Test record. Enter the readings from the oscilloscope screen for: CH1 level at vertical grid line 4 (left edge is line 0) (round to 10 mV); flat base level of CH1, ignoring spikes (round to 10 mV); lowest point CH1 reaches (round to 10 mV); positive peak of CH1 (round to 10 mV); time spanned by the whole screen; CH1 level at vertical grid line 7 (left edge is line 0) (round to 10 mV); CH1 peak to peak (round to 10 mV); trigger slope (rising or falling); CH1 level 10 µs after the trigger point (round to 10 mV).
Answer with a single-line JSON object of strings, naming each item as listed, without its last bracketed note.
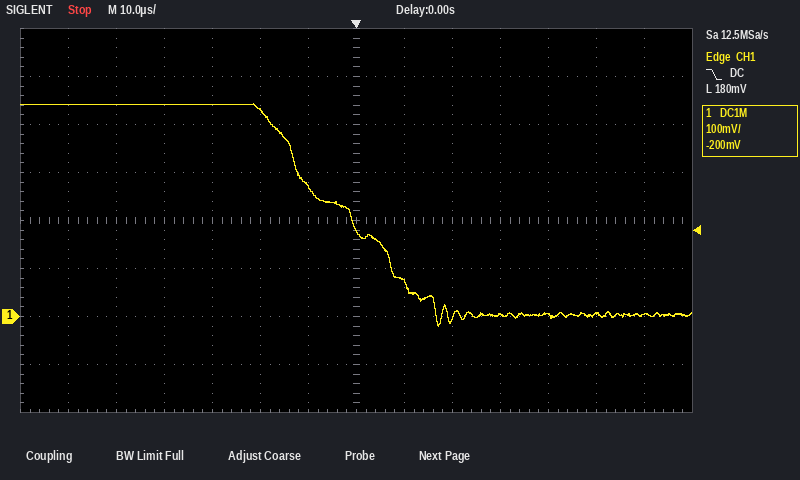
{"CH1 level at vertical grid line 4 (left edge is line 0)": "440 mV", "flat base level of CH1, ignoring spikes": "0 mV", "lowest point CH1 reaches": "-20 mV", "positive peak of CH1": "440 mV", "time spanned by the whole screen": "140 µs", "CH1 level at vertical grid line 7 (left edge is line 0)": "180 mV", "CH1 peak to peak": "460 mV", "trigger slope": "falling", "CH1 level 10 µs after the trigger point": "70 mV"}
